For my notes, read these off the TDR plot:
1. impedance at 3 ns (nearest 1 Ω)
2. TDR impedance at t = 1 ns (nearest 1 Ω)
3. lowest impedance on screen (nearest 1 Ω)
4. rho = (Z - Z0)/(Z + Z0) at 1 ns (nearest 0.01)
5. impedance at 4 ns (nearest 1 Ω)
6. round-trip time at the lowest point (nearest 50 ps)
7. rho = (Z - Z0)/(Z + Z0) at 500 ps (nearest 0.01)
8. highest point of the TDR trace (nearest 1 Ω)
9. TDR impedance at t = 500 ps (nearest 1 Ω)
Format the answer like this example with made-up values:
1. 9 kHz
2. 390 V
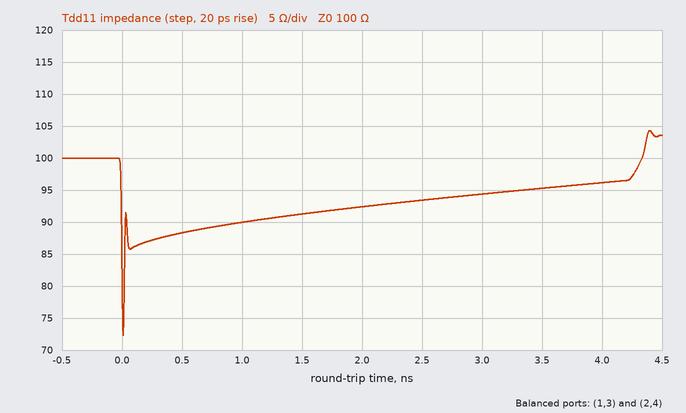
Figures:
1. 94 Ω
2. 90 Ω
3. 72 Ω
4. -0.05
5. 96 Ω
6. 0 ps
7. -0.06
8. 104 Ω
9. 88 Ω
